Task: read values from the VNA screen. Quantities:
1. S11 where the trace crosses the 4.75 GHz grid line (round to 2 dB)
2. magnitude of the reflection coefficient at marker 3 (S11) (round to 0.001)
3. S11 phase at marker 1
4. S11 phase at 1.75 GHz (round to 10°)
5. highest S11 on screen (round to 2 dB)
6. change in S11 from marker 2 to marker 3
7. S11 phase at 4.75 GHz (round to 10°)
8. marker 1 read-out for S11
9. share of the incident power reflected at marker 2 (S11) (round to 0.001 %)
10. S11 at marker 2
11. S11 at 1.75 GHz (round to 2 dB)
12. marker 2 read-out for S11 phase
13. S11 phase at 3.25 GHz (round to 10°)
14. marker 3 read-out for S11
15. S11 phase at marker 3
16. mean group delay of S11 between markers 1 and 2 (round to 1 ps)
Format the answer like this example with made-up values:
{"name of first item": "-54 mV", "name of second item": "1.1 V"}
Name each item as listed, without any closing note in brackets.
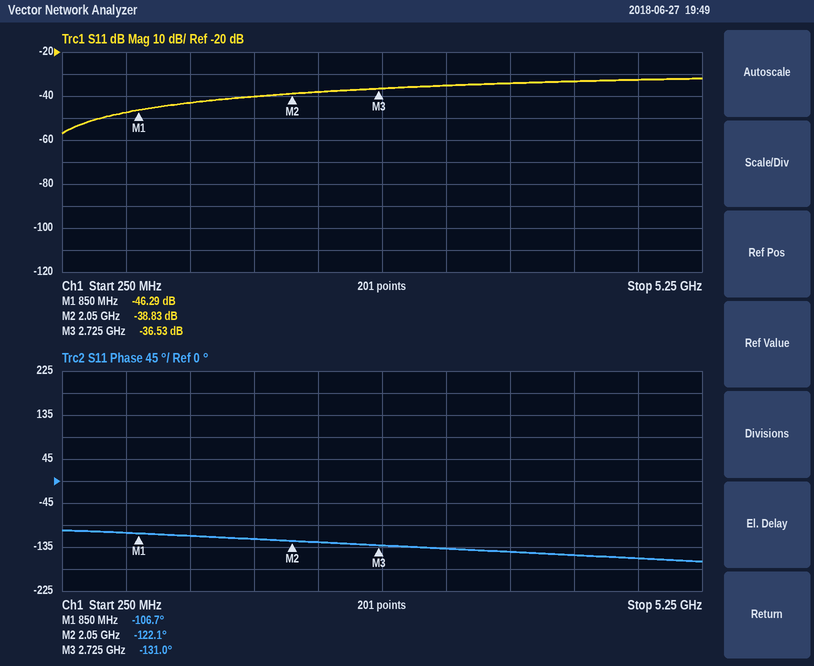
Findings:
{"S11 where the trace crosses the 4.75 GHz grid line": "-32 dB", "magnitude of the reflection coefficient at marker 3 (S11)": "0.015", "S11 phase at marker 1": "-106.7°", "S11 phase at 1.75 GHz": "-120°", "highest S11 on screen": "-32 dB", "change in S11 from marker 2 to marker 3": "2.30 dB", "S11 phase at 4.75 GHz": "-160°", "marker 1 read-out for S11": "-46.29 dB", "share of the incident power reflected at marker 2 (S11)": "0.013 %", "S11 at marker 2": "-38.83 dB", "S11 at 1.75 GHz": "-40 dB", "marker 2 read-out for S11 phase": "-122.1°", "S11 phase at 3.25 GHz": "-140°", "marker 3 read-out for S11": "-36.53 dB", "S11 phase at marker 3": "-131.0°", "mean group delay of S11 between markers 1 and 2": "36 ps"}
